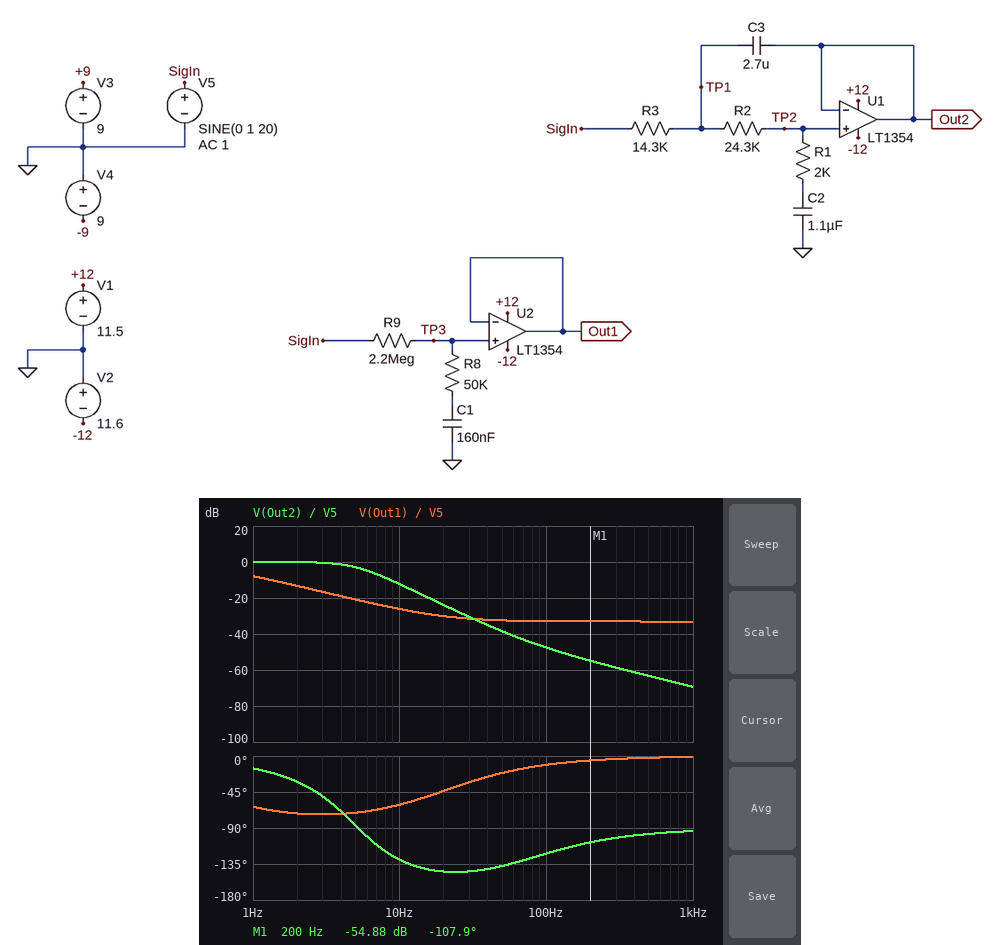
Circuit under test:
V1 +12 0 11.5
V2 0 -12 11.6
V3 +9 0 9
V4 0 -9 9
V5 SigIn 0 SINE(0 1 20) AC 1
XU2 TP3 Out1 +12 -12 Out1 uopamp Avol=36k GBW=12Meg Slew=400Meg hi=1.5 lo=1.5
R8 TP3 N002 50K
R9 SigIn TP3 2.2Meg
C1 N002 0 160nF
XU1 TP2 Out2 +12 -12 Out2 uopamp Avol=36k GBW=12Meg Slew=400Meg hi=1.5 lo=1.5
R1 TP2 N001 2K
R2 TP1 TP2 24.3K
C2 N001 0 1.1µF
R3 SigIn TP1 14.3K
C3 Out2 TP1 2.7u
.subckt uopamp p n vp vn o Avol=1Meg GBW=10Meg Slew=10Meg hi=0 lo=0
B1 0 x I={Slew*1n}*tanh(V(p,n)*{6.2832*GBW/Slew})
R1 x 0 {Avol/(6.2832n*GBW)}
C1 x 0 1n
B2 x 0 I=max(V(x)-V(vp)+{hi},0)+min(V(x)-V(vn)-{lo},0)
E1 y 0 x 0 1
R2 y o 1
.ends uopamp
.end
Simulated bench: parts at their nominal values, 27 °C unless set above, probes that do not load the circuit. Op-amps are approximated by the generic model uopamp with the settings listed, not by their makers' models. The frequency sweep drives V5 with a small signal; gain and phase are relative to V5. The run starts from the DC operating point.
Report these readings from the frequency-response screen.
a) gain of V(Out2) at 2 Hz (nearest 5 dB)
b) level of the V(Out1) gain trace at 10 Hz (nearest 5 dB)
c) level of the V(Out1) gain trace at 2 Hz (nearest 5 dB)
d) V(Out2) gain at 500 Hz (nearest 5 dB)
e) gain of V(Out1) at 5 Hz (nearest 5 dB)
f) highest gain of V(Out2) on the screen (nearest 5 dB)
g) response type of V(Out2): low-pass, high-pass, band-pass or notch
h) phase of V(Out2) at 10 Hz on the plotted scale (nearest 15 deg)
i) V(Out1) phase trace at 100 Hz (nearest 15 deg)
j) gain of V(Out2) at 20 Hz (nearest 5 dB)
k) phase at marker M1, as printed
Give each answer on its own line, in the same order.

0 dB
-25 dB
-15 dB
-65 dB
-20 dB
0 dB
low-pass
-135 deg
-15 deg
-25 dB
-107.9 deg
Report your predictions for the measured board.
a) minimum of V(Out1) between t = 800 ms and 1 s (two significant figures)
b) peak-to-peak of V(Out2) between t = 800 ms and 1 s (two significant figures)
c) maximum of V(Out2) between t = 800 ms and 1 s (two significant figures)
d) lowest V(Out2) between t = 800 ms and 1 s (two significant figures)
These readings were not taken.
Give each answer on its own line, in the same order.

-30 mV
130 mV
64 mV
-64 mV
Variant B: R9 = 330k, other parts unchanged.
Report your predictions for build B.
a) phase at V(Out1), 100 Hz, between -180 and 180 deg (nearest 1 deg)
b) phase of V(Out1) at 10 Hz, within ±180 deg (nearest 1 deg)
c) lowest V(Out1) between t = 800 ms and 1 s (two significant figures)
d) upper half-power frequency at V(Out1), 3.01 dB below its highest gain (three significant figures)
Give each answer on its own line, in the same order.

-10 deg
-49 deg
-180 mV
2.66 Hz
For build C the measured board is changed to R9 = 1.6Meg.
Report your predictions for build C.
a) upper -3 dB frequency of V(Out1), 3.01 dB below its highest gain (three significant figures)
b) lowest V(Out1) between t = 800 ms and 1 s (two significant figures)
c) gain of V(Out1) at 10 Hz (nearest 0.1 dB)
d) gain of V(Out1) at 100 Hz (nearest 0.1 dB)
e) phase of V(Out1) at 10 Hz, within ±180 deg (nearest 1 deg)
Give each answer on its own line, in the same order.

603 mHz
-42 mV
-23.4 dB
-30.2 dB
-60 deg
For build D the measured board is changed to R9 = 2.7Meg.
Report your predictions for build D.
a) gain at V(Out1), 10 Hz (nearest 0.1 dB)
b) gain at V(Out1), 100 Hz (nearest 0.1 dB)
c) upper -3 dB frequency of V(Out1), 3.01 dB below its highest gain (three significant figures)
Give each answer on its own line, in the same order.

-27.9 dB
-34.6 dB
362 mHz
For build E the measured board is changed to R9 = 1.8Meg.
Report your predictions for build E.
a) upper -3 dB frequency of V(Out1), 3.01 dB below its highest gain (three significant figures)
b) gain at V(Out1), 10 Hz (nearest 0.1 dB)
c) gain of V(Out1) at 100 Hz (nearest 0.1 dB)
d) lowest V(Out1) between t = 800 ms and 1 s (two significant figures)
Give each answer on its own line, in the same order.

538 mHz
-24.4 dB
-31.2 dB
-37 mV
